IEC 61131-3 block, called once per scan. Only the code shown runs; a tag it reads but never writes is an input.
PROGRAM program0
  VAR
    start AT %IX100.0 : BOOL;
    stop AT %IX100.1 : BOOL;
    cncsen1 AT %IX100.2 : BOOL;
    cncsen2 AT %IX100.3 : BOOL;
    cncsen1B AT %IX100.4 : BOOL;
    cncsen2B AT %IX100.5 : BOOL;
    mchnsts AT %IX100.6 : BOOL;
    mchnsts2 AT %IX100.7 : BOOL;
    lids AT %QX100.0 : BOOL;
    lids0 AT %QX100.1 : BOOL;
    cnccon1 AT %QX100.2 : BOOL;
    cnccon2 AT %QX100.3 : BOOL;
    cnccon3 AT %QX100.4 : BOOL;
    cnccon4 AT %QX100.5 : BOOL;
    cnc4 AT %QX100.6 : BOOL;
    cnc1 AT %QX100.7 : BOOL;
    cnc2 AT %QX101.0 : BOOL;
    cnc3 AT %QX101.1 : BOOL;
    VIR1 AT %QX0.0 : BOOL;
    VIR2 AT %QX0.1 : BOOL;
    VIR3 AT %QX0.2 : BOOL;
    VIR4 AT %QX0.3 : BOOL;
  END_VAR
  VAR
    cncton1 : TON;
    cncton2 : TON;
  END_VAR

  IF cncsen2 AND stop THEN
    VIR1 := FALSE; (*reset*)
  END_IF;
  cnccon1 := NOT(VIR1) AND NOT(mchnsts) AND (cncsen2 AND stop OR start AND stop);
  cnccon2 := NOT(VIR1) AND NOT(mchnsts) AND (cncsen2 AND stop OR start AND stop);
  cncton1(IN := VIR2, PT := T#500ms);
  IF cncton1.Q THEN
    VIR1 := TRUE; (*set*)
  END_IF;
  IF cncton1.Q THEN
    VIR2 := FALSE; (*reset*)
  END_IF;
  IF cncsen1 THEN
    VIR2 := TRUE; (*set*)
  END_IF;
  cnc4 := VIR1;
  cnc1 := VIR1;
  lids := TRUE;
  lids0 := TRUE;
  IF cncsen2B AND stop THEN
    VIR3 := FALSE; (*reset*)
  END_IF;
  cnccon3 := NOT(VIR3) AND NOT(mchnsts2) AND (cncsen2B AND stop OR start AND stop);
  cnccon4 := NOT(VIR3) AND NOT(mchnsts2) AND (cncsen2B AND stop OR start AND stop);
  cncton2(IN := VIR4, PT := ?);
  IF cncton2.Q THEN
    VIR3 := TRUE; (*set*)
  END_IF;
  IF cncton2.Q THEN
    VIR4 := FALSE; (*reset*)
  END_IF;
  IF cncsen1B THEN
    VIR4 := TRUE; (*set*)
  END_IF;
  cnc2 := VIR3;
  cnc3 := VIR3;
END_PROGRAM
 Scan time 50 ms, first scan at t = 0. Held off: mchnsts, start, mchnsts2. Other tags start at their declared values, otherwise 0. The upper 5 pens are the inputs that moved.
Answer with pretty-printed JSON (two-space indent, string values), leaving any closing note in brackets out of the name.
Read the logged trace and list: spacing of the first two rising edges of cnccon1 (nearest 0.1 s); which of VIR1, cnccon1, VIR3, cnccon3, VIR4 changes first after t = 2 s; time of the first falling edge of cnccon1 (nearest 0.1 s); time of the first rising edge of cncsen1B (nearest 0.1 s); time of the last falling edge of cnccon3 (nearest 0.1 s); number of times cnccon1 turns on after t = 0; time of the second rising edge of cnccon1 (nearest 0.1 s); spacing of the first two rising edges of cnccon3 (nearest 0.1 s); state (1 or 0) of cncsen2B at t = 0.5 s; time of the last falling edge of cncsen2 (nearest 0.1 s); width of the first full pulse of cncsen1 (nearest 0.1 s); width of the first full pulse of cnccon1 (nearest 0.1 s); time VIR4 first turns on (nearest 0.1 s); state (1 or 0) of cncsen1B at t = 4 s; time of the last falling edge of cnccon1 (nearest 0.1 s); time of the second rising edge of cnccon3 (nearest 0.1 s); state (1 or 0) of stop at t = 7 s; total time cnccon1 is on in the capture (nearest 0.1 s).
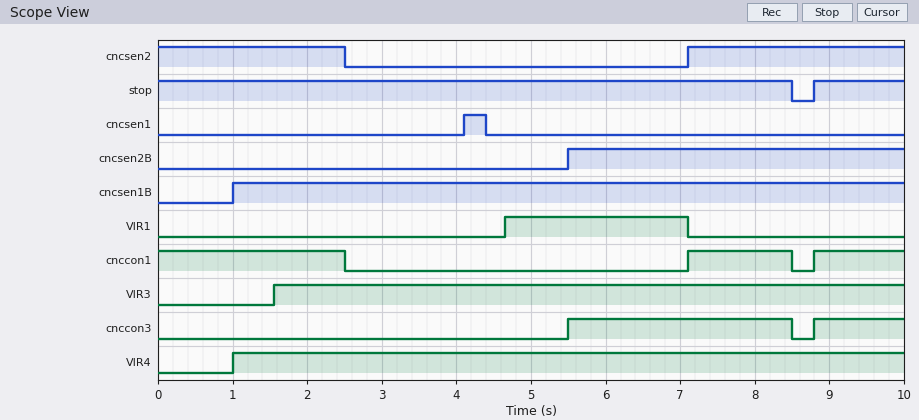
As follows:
{
  "spacing of the first two rising edges of cnccon1": "1.7 s",
  "which of VIR1, cnccon1, VIR3, cnccon3, VIR4 changes first after t = 2 s": "cnccon1",
  "time of the first falling edge of cnccon1": "2.5 s",
  "time of the first rising edge of cncsen1B": "1.0 s",
  "time of the last falling edge of cnccon3": "8.5 s",
  "number of times cnccon1 turns on after t = 0": "2",
  "time of the second rising edge of cnccon1": "8.8 s",
  "spacing of the first two rising edges of cnccon3": "3.3 s",
  "state (1 or 0) of cncsen2B at t = 0.5 s": "0",
  "time of the last falling edge of cncsen2": "2.5 s",
  "width of the first full pulse of cncsen1": "0.3 s",
  "width of the first full pulse of cnccon1": "1.4 s",
  "time VIR4 first turns on": "1.0 s",
  "state (1 or 0) of cncsen1B at t = 4 s": "1",
  "time of the last falling edge of cnccon1": "8.5 s",
  "time of the second rising edge of cnccon3": "8.8 s",
  "state (1 or 0) of stop at t = 7 s": "1",
  "total time cnccon1 is on in the capture": "5.1 s"
}
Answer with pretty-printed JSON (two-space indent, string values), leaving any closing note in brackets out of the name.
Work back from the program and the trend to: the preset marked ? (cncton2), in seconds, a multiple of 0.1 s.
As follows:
{
  "the preset marked ? (cncton2), in seconds, a multiple of 0.1 s": "0.5 s"
}
